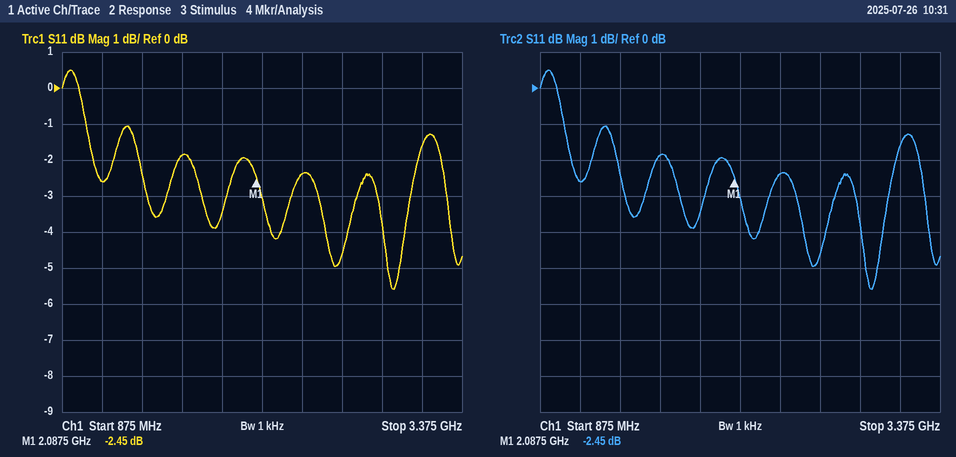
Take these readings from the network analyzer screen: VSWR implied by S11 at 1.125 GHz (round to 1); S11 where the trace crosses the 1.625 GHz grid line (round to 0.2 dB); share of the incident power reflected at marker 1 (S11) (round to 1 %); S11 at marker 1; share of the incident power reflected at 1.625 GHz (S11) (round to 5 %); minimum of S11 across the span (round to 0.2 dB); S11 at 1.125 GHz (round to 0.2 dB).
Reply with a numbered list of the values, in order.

1. 7
2. -1.8 dB
3. 57 %
4. -2.45 dB
5. 65 %
6. -5.6 dB
7. -2.6 dB
